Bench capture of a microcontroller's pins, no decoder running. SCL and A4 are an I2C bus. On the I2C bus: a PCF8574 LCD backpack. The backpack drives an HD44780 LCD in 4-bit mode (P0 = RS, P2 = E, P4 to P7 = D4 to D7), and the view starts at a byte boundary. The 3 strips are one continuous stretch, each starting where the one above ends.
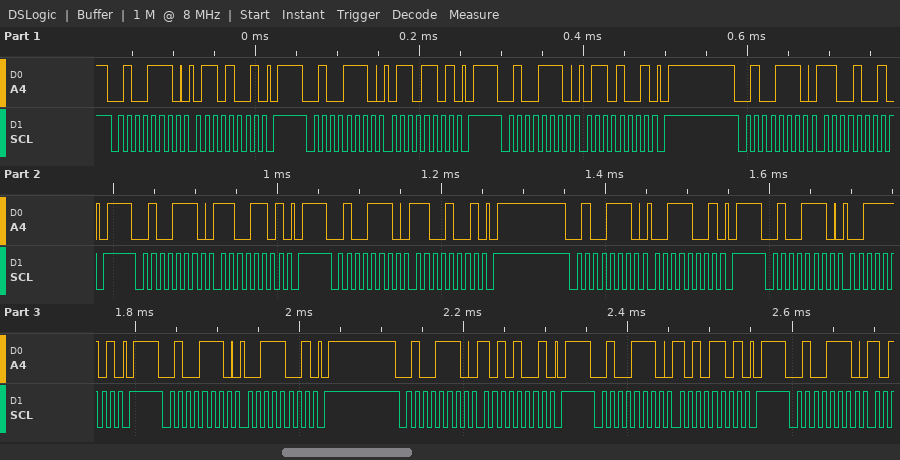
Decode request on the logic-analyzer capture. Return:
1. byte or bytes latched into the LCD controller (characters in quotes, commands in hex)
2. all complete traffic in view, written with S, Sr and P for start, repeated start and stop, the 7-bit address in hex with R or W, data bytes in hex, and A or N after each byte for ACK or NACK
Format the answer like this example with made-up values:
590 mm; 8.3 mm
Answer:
'l'; S 27W A 69 A P S 27W A 6D A P S 27W A 69 A P S 27W A C9 A P S 27W A CD A P S 27W A C9 A P S 27W A 39 A P S 27W A 3D A P S 27W A 39 A P S 27W A A9 A P S 27W A AD A P S 27W A
